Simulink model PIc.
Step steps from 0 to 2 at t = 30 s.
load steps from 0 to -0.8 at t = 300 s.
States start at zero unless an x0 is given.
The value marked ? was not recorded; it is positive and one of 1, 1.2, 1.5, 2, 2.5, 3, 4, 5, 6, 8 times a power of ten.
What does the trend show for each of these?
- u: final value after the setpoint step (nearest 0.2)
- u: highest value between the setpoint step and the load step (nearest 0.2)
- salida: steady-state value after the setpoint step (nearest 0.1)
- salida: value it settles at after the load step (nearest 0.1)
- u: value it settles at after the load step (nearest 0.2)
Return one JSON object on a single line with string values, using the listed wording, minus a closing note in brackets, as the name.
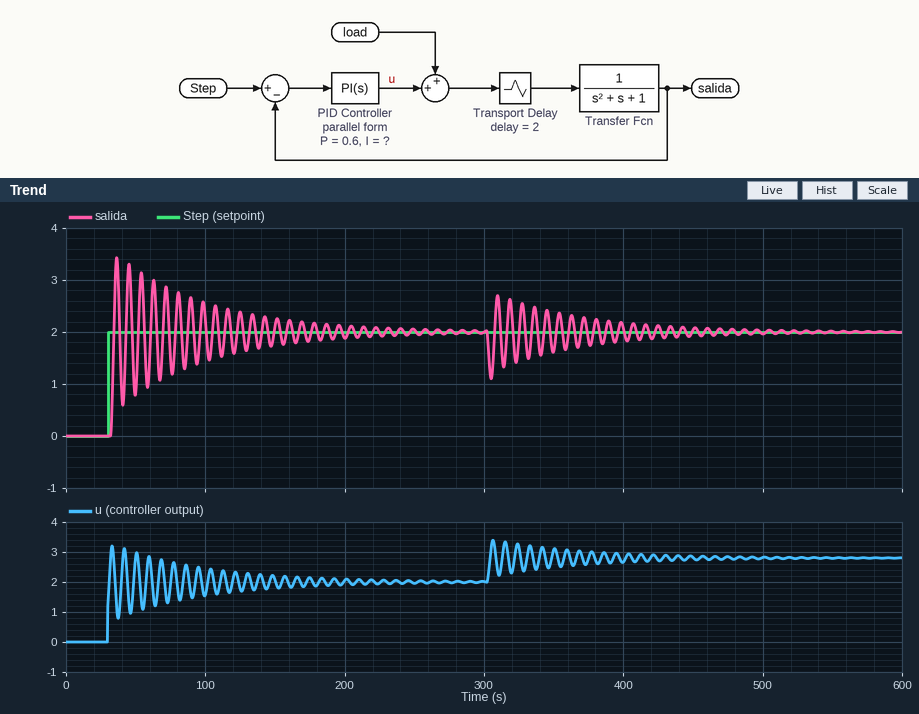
{"u: final value after the setpoint step": "2.0", "u: highest value between the setpoint step and the load step": "3.2", "salida: steady-state value after the setpoint step": "2.0", "salida: value it settles at after the load step": "2.0", "u: value it settles at after the load step": "2.8"}
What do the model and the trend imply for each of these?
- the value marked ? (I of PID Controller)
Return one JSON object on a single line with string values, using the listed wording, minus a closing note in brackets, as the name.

{"the value marked ?": "0.4"}
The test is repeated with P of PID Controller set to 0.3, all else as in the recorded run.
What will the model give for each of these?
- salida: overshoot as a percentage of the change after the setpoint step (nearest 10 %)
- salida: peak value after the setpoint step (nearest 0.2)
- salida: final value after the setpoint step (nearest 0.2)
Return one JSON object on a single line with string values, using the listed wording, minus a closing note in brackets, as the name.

{"salida: overshoot as a percentage of the change after the setpoint step": "70 %", "salida: peak value after the setpoint step": "3.4", "salida: final value after the setpoint step": "2.0"}
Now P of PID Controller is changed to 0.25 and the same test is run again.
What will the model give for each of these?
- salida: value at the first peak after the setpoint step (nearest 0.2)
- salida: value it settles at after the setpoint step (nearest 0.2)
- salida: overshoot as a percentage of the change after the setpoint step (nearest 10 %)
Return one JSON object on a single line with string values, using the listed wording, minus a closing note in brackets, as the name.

{"salida: value at the first peak after the setpoint step": "3.4", "salida: value it settles at after the setpoint step": "2.0", "salida: overshoot as a percentage of the change after the setpoint step": "70 %"}
